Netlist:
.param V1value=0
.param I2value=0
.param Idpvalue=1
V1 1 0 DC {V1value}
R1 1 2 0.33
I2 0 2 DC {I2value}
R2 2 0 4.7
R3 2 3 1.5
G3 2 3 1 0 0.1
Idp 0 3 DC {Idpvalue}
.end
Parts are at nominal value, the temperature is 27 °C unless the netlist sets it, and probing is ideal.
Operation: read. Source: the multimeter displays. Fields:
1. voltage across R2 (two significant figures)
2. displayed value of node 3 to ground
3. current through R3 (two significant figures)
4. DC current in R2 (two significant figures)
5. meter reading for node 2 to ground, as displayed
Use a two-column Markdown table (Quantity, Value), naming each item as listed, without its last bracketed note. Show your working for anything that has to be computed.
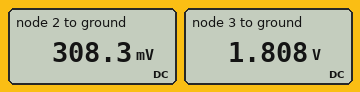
| Quantity | Value |
|---|---|
| voltage across R2 | 308.3 mV = 310 mV |
| displayed value of node 3 to ground | 1.808 V |
| current through R3 | (1.808 V - 308.3 mV) / 1.5 Ω = 1.0 A |
| DC current in R2 | (308.3 mV) / 4.7 Ω = 66 mA |
| meter reading for node 2 to ground, as displayed | 308.3 mV |
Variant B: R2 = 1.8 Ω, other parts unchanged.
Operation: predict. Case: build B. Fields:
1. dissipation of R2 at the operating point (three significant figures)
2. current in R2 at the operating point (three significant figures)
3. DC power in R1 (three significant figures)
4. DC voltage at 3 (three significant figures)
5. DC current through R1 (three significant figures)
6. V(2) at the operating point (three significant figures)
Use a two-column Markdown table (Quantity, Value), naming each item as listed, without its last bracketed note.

| Quantity | Value |
|---|---|
| dissipation of R2 at the operating point | 43.2 mW |
| current in R2 at the operating point | 155 mA |
| DC power in R1 | 236 mW |
| DC voltage at 3 | 1.78 V |
| DC current through R1 | 845 mA |
| V(2) at the operating point | 279 mV |
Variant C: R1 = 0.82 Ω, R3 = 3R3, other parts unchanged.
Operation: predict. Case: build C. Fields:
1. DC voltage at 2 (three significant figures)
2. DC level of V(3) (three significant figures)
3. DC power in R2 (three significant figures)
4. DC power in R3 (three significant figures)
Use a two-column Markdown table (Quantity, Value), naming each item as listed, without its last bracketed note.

| Quantity | Value |
|---|---|
| DC voltage at 2 | 698 mV |
| DC level of V(3) | 4.00 V |
| DC power in R2 | 104 mW |
| DC power in R3 | 3.30 W |
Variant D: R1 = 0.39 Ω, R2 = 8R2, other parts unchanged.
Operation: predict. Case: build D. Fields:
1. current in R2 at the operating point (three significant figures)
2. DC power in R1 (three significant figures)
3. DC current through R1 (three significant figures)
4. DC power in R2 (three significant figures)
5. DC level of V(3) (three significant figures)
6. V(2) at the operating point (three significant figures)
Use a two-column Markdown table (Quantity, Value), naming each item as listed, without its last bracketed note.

| Quantity | Value |
|---|---|
| current in R2 at the operating point | 45.4 mA |
| DC power in R1 | 355 mW |
| DC current through R1 | 955 mA |
| DC power in R2 | 16.9 mW |
| DC level of V(3) | 1.87 V |
| V(2) at the operating point | 372 mV |
